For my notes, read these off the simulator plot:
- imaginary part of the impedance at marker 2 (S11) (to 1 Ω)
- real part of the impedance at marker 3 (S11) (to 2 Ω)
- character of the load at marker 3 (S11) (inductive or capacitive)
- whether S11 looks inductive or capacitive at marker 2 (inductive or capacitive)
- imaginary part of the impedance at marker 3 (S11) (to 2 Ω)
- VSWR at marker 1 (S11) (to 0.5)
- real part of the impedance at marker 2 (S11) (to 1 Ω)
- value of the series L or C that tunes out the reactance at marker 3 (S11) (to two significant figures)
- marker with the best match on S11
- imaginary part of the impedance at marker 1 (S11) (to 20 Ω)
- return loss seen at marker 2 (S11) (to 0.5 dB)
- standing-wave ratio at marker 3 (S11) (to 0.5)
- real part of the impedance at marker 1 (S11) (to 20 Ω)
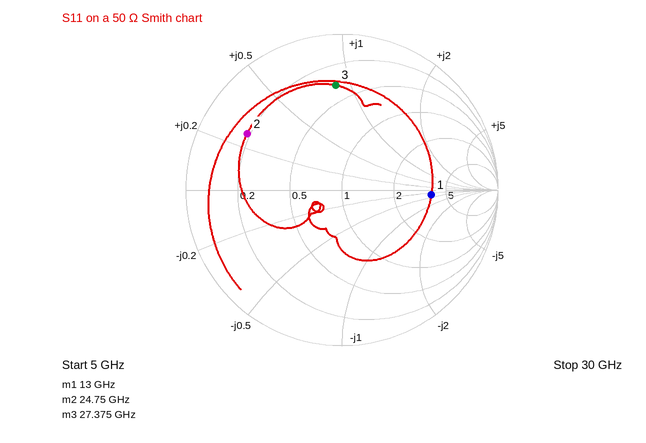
+13 Ω
18 Ω
inductive
inductive
+44 Ω
3.5
9 Ω
130 fF
marker 1
-20 Ω
3.0 dB
5.0
180 Ω
